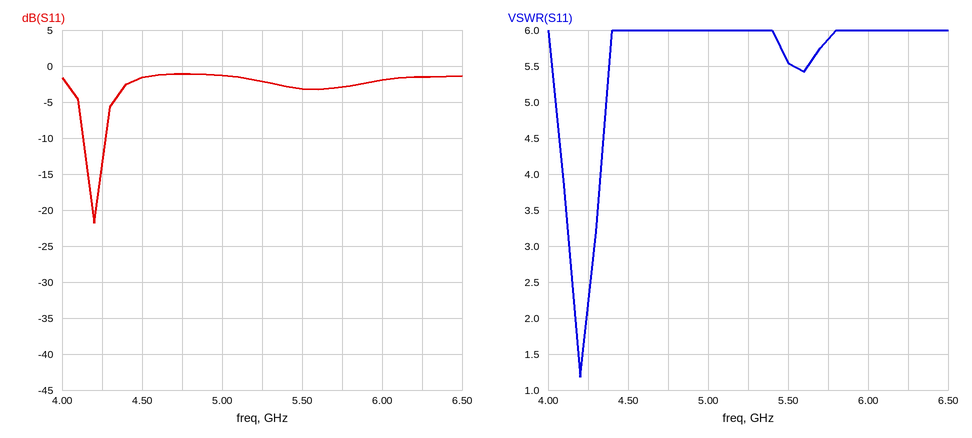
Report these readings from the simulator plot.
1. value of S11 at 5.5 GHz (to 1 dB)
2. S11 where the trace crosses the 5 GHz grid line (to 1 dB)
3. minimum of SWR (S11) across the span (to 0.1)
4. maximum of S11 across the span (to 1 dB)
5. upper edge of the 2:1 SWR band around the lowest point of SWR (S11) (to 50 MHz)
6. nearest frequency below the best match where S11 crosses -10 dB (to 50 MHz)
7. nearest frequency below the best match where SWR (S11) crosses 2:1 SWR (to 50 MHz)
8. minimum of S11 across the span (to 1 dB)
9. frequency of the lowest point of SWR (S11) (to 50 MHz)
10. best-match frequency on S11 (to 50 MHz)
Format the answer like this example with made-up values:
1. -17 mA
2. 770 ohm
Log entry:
1. -3 dB
2. -1 dB
3. 1.2
4. -1 dB
5. 4.25 GHz
6. 4.15 GHz
7. 4.15 GHz
8. -22 dB
9. 4.20 GHz
10. 4.20 GHz
